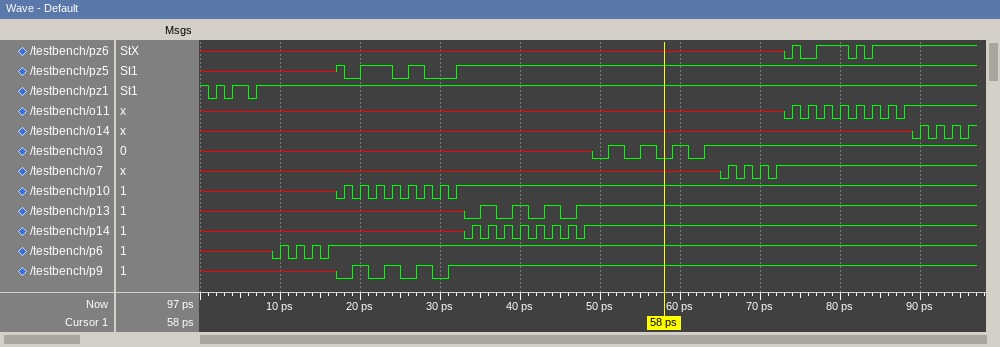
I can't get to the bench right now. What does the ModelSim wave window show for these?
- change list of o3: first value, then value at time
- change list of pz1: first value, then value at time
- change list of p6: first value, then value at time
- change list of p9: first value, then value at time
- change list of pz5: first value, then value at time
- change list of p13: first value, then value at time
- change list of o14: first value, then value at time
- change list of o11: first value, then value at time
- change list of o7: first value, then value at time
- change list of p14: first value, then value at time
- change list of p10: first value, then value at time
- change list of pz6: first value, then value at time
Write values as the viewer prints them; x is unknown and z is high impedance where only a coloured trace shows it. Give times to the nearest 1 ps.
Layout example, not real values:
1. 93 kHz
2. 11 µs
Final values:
1. x, 0 at 49 ps, 1 at 51 ps, 0 at 53 ps, 1 at 55 ps, 0 at 57 ps, 1 at 59 ps, 0 at 61 ps, 1 at 63 ps
2. 1, 0 at 1 ps, 1 at 2 ps, 0 at 3 ps, 1 at 4 ps, 0 at 6 ps, 1 at 7 ps
3. x, 0 at 9 ps, 1 at 10 ps, 0 at 11 ps, 1 at 12 ps, 0 at 13 ps, 1 at 14 ps, 0 at 15 ps, 1 at 16 ps
4. x, 0 at 17 ps, 1 at 19 ps, 0 at 21 ps, 1 at 23 ps, 0 at 25 ps, 1 at 27 ps, 0 at 29 ps, 1 at 31 ps
5. x, 1 at 17 ps, 0 at 18 ps, 1 at 20 ps, 0 at 24 ps, 1 at 26 ps, 0 at 28 ps, 1 at 32 ps
6. x, 0 at 33 ps, 1 at 35 ps, 0 at 37 ps, 1 at 39 ps, 0 at 41 ps, 1 at 43 ps, 0 at 45 ps, 1 at 47 ps
7. x, 0 at 89 ps, 1 at 90 ps, 0 at 91 ps, 1 at 92 ps, 0 at 93 ps, 1 at 94 ps, 0 at 95 ps, 1 at 96 ps
8. x, 0 at 73 ps, 1 at 74 ps, 0 at 75 ps, 1 at 76 ps, 0 at 77 ps, 1 at 78 ps, 0 at 79 ps, 1 at 80 ps, 0 at 81 ps, 1 at 82 ps, 0 at 83 ps, 1 at 84 ps, 0 at 85 ps, 1 at 86 ps, 0 at 87 ps, 1 at 88 ps
9. x, 0 at 65 ps, 1 at 66 ps, 0 at 67 ps, 1 at 68 ps, 0 at 69 ps, 1 at 70 ps, 0 at 71 ps, 1 at 72 ps
10. x, 0 at 33 ps, 1 at 34 ps, 0 at 35 ps, 1 at 36 ps, 0 at 37 ps, 1 at 38 ps, 0 at 39 ps, 1 at 40 ps, 0 at 41 ps, 1 at 42 ps, 0 at 43 ps, 1 at 44 ps, 0 at 45 ps, 1 at 46 ps, 0 at 47 ps, 1 at 48 ps
11. x, 0 at 17 ps, 1 at 18 ps, 0 at 19 ps, 1 at 20 ps, 0 at 21 ps, 1 at 22 ps, 0 at 23 ps, 1 at 24 ps, 0 at 25 ps, 1 at 26 ps, 0 at 27 ps, 1 at 28 ps, 0 at 29 ps, 1 at 30 ps, 0 at 31 ps, 1 at 32 ps
12. x, 0 at 73 ps, 1 at 74 ps, 0 at 75 ps, 1 at 77 ps, 0 at 81 ps, 1 at 82 ps, 0 at 83 ps, 1 at 84 ps
